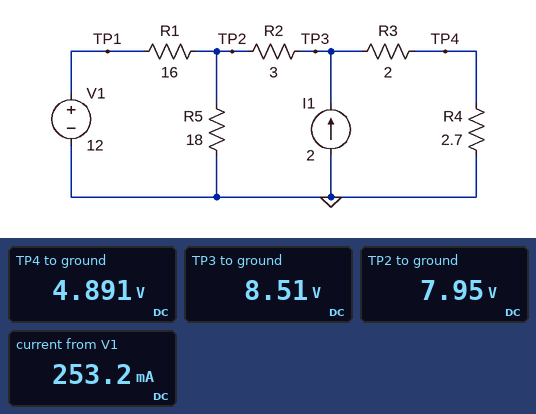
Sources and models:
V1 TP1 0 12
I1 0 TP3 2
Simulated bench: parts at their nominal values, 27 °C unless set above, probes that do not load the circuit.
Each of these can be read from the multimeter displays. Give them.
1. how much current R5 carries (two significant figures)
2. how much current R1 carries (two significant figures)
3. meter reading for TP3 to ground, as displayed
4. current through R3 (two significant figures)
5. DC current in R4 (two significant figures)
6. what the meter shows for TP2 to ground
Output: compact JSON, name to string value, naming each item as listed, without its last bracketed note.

{"how much current R5 carries": "440 mA", "how much current R1 carries": "250 mA", "meter reading for TP3 to ground, as displayed": "8.51 V", "current through R3": "1.8 A", "DC current in R4": "1.8 A", "what the meter shows for TP2 to ground": "7.95 V"}
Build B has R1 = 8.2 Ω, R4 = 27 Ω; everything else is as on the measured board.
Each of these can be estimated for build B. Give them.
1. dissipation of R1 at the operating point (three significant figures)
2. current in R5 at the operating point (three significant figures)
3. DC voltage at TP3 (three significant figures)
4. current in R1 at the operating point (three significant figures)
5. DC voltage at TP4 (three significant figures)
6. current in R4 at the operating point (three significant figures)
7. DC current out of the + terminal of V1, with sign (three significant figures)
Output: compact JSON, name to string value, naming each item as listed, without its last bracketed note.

{"dissipation of R1 at the operating point": "1.66 W", "current in R5 at the operating point": "872 mA", "DC voltage at TP3": "19.7 V", "current in R1 at the operating point": "450 mA", "DC voltage at TP4": "18.3 V", "current in R4 at the operating point": "678 mA", "DC current out of the + terminal of V1, with sign": "-450 mA"}
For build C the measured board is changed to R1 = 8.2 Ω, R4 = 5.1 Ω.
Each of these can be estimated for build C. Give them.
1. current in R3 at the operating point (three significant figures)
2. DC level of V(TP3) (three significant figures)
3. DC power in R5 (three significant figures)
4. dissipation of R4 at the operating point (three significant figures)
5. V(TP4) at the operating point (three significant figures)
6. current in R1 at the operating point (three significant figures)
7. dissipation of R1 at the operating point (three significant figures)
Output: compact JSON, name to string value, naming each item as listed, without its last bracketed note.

{"current in R3 at the operating point": "1.62 A", "DC level of V(TP3)": "11.5 V", "DC power in R5": "5.98 W", "dissipation of R4 at the operating point": "13.4 W", "V(TP4) at the operating point": "8.27 V", "current in R1 at the operating point": "198 mA", "dissipation of R1 at the operating point": "321 mW"}
